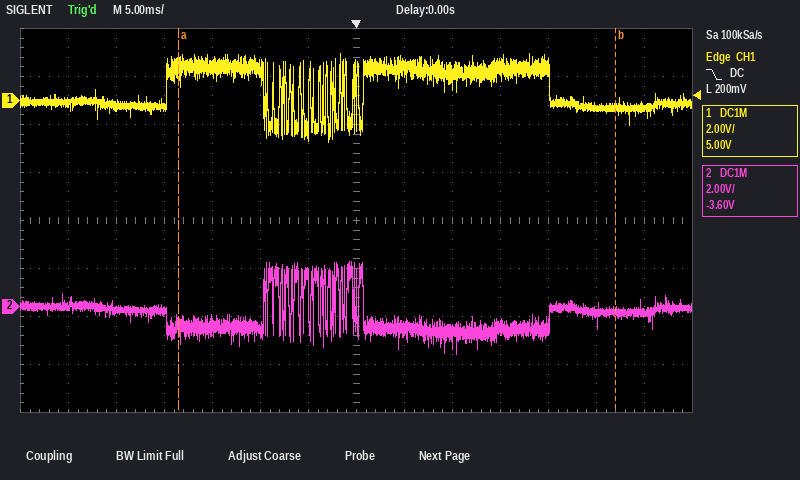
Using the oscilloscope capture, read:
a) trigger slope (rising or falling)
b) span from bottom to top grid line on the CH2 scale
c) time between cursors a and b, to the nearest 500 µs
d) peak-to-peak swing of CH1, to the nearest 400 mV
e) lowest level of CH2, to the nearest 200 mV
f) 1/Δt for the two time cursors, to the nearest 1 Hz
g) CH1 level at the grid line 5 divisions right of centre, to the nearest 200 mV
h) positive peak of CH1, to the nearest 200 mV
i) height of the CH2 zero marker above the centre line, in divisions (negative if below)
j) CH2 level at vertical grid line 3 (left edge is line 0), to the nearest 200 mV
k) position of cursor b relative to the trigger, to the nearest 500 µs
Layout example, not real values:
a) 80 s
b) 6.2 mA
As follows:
a) falling
b) 16 V
c) 45.5 ms
d) 3.6 V
e) -2.0 V
f) 22 Hz
g) -200 mV
h) 2.0 V
i) -1.8 div
j) -200 mV
k) +27.0 ms
